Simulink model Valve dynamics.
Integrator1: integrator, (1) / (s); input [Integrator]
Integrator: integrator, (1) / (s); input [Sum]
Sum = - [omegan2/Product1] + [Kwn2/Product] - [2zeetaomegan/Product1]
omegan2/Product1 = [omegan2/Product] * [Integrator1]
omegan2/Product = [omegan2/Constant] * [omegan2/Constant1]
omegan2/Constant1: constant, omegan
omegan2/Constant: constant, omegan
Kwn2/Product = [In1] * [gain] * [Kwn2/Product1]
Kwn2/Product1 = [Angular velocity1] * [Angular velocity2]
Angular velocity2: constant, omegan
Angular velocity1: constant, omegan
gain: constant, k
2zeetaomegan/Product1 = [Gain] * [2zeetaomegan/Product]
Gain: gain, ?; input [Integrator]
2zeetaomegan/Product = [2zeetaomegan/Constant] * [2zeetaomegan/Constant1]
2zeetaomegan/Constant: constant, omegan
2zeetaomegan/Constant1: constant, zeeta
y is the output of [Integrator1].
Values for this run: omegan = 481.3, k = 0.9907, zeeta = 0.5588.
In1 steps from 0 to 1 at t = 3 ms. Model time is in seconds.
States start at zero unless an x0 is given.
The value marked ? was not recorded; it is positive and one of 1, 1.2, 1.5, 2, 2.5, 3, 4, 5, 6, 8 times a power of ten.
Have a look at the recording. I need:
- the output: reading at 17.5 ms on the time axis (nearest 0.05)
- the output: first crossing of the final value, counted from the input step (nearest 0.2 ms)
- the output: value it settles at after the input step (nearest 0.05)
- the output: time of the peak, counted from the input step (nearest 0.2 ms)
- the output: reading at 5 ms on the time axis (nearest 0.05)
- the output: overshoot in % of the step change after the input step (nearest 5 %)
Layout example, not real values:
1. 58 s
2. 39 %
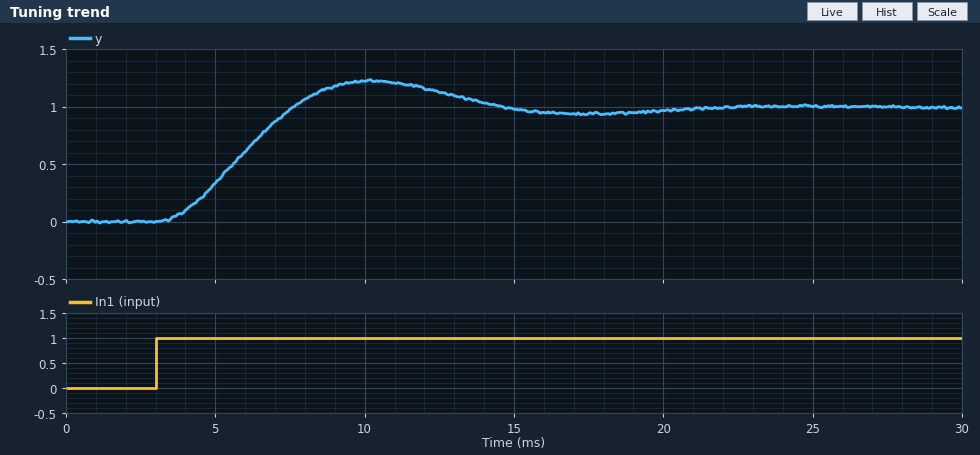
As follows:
1. 0.95
2. 4.6 ms
3. 1.00
4. 7.2 ms
5. 0.35
6. 25 %
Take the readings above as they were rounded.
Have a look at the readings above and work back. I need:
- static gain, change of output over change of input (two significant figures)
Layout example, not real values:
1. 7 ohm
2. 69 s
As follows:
1. 1.0
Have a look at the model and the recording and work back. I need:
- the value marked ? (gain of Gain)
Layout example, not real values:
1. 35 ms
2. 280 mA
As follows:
1. 1.5
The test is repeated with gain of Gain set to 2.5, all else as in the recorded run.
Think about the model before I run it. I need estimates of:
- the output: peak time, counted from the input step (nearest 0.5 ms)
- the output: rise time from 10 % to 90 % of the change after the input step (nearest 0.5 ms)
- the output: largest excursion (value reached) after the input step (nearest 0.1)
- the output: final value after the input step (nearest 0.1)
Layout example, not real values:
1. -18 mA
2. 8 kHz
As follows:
1. 9.0 ms
2. 4.5 ms
3. 1.0
4. 1.0
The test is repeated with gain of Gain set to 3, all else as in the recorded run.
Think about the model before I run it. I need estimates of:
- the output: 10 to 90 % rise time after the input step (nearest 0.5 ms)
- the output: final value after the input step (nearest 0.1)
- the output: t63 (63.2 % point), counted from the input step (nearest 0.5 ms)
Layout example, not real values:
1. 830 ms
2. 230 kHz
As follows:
1. 5.5 ms
2. 1.0
3. 4.0 ms
